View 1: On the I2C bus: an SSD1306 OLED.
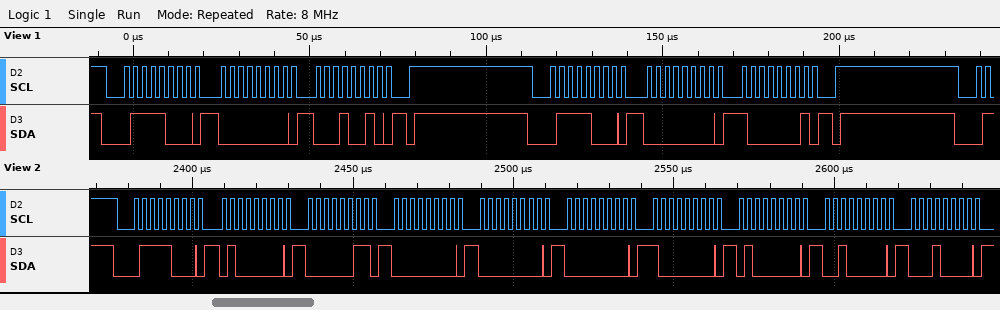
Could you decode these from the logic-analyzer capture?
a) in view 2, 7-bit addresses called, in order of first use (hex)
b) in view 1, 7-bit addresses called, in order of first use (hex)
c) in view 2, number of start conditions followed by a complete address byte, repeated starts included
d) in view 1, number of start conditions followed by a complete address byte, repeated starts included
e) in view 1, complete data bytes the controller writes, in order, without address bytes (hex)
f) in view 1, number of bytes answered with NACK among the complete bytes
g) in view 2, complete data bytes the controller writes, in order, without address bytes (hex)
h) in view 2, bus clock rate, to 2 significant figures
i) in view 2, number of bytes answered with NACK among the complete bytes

0x3C
0x3C
1
2
00 12 00 81
0
40 03 00 00 00 80 40 20 10
400 kHz
0
